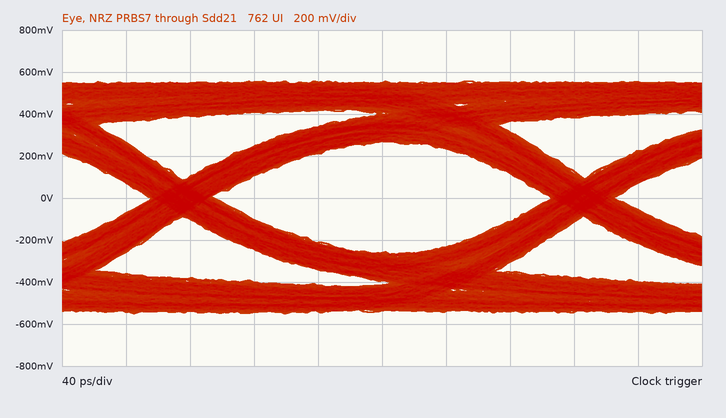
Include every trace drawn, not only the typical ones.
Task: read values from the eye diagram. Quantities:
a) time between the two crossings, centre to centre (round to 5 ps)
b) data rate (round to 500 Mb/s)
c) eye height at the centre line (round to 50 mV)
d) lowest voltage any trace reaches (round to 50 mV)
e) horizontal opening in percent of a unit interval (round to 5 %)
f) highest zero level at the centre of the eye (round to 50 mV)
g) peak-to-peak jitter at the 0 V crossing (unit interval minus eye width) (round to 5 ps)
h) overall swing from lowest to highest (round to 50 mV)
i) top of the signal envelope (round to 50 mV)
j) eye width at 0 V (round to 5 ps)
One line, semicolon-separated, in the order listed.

250 ps; 4.0 Gb/s; 550 mV; -550 mV; 85 %; -250 mV; 40 ps; 1.10 V; 550 mV; 210 ps
